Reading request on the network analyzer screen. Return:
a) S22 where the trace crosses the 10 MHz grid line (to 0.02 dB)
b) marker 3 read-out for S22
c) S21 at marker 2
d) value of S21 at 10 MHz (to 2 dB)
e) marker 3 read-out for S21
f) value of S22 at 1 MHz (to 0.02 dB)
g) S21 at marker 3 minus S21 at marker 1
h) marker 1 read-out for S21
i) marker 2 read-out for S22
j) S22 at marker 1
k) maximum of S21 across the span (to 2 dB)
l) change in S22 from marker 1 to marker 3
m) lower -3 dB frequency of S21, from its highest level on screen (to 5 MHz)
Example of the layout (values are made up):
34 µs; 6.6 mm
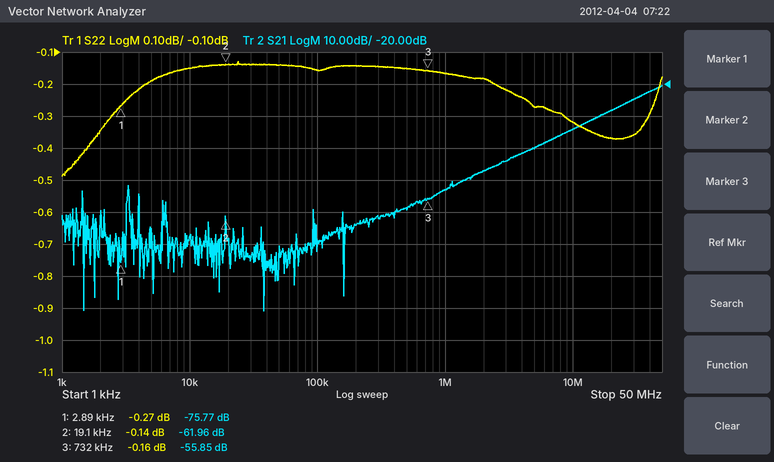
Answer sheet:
-0.32 dB; -0.16 dB; -61.96 dB; -34 dB; -55.85 dB; -0.16 dB; 19.92 dB; -75.77 dB; -0.14 dB; -0.27 dB; -20 dB; 0.11 dB; 35 MHz
